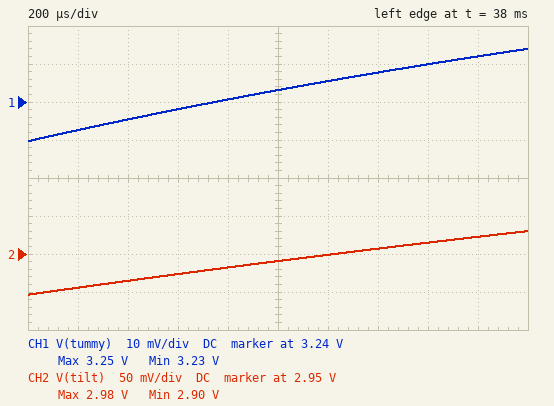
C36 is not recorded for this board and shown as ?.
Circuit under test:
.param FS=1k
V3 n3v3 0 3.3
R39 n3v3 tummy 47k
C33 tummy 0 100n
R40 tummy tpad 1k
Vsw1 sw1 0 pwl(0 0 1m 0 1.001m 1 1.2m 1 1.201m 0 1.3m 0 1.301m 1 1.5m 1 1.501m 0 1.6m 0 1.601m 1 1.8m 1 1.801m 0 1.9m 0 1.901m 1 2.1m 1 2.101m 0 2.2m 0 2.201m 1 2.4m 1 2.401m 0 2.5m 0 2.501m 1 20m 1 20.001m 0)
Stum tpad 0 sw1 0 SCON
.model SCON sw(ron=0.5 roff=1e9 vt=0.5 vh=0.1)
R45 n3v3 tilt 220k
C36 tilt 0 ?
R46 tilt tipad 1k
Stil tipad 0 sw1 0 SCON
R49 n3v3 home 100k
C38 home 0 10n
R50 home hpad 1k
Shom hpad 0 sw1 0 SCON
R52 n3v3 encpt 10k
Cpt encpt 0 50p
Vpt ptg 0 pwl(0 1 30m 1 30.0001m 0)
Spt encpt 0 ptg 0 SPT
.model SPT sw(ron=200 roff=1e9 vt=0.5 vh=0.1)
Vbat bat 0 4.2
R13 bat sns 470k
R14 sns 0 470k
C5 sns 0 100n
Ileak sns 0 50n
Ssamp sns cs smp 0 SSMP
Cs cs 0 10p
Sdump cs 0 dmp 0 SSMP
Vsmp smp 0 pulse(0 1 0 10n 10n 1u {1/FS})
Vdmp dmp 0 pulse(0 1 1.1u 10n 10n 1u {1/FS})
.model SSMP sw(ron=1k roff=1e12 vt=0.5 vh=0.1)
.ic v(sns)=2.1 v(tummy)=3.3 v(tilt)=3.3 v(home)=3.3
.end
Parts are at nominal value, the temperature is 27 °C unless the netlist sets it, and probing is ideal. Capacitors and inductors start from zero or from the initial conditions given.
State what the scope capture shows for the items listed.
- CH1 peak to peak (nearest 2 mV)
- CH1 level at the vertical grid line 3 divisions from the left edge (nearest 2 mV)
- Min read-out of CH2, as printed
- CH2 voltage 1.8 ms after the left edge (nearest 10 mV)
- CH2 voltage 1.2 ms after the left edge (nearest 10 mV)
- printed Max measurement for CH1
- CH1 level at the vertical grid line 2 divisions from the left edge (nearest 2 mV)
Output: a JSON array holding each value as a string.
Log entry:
["24 mV", "3.238 V", "2.90 V", "2.97 V", "2.95 V", "3.25 V", "3.236 V"]
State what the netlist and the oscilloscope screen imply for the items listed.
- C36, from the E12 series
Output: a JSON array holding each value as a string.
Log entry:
["39 nF"]
